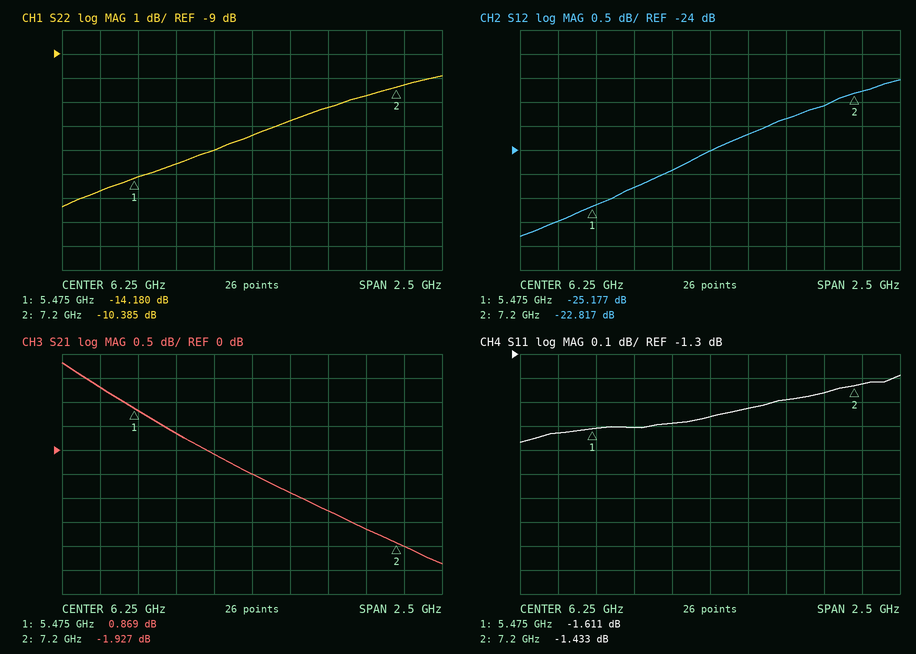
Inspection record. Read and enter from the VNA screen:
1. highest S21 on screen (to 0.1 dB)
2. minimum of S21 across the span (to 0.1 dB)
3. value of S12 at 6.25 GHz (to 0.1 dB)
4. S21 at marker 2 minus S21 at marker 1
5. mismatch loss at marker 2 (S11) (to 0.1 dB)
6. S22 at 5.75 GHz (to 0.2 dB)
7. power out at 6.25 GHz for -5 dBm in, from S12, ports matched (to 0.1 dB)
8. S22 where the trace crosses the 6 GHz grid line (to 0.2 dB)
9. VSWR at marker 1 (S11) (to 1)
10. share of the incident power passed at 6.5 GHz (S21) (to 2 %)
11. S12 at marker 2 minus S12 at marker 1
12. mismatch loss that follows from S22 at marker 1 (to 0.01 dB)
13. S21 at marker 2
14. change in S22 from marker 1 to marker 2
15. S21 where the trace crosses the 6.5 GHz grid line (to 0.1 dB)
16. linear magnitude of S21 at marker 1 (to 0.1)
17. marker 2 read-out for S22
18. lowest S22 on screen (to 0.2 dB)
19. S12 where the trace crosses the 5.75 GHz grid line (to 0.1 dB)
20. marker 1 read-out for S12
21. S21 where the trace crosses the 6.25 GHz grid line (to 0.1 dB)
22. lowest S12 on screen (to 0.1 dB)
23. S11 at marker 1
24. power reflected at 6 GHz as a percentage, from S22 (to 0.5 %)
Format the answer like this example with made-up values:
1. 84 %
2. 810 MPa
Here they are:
1. 1.8 dB
2. -2.4 dB
3. -24.0 dB
4. -2.796 dB
5. 5.5 dB
6. -13.6 dB
7. -29.0 dBm
8. -13.0 dB
9. 11
10. 82 %
11. 2.360 dB
12. 0.17 dB
13. -1.927 dB
14. 3.795 dB
15. -0.9 dB
16. 1.1
17. -10.385 dB
18. -15.4 dB
19. -24.8 dB
20. -25.177 dB
21. -0.5 dB
22. -25.8 dB
23. -1.611 dB
24. 5.0 %
